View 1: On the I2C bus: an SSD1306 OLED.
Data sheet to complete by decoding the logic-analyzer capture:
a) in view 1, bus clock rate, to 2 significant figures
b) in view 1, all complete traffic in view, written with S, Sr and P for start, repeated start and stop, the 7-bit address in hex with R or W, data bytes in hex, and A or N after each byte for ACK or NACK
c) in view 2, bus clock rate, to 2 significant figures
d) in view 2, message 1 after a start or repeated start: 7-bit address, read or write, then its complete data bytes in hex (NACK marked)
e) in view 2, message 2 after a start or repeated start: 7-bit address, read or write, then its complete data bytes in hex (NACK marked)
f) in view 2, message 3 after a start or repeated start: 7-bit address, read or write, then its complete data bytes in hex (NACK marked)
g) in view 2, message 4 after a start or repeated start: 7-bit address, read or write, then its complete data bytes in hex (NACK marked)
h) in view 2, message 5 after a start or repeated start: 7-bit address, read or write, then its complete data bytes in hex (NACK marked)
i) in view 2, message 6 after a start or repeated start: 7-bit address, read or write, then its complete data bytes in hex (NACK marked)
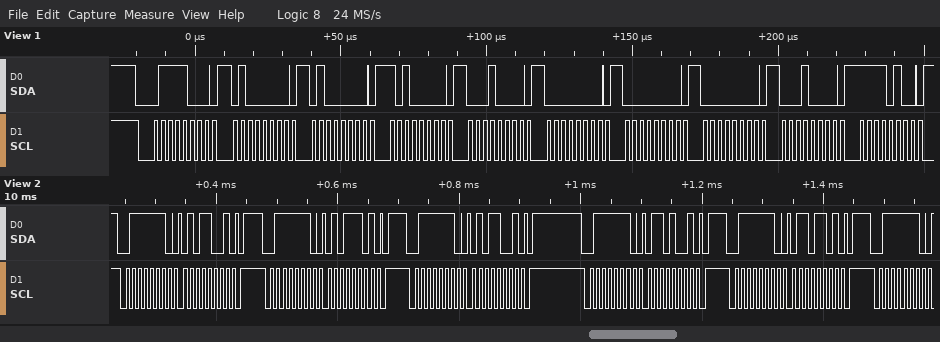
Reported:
400 kHz
S 3CW A 40 A 40 A A0 A 10 A 00 A 00 A 00 A 10 A F4 A
100 kHz
0x3F write: 59
0x3F write: 5D
0x3F write: 59
0x3F write: 69
0x3F write: 6D
0x3F write
